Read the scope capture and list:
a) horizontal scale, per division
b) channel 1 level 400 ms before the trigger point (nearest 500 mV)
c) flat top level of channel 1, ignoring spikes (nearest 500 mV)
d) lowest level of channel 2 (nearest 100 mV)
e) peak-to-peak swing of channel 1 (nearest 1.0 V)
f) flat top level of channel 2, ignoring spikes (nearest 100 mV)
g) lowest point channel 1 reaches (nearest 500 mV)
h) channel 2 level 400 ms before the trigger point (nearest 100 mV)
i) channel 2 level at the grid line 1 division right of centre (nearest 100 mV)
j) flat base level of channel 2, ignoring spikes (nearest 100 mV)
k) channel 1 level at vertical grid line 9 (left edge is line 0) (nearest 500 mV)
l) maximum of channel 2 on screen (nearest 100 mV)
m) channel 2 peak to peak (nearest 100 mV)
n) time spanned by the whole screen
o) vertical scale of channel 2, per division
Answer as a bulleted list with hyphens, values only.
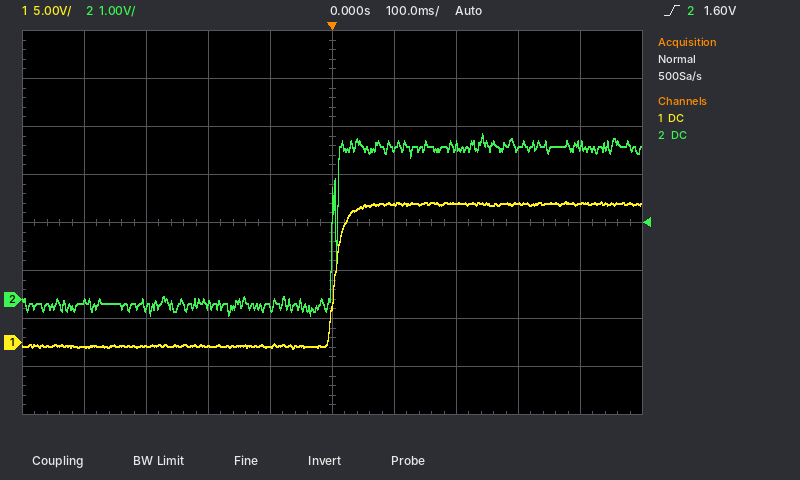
- 100 ms
- -500 mV
- 14.5 V
- -300 mV
- 15.0 V
- 3.2 V
- -500 mV
- 0.0 V
- 3.1 V
- -100 mV
- 14.5 V
- 3.5 V
- 3.8 V
- 1 s
- 1 V
